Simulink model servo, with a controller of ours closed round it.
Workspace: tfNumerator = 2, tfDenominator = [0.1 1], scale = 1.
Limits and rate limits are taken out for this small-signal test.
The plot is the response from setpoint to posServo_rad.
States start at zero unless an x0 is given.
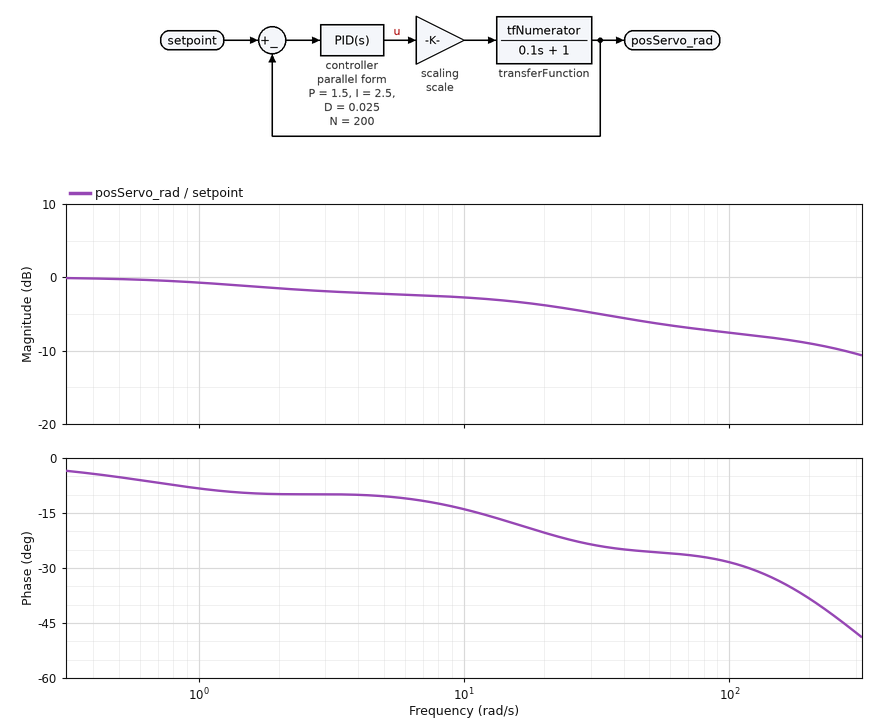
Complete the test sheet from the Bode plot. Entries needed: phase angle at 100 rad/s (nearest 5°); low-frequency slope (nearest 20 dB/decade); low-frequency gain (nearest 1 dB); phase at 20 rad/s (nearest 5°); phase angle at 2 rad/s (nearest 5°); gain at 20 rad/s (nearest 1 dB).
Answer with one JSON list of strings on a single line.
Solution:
["-30°", "0 dB/decade", "0 dB", "-20°", "-10°", "-4 dB"]
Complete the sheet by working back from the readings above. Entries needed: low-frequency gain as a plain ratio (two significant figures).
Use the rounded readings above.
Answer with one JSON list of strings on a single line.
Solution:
["1.0"]
